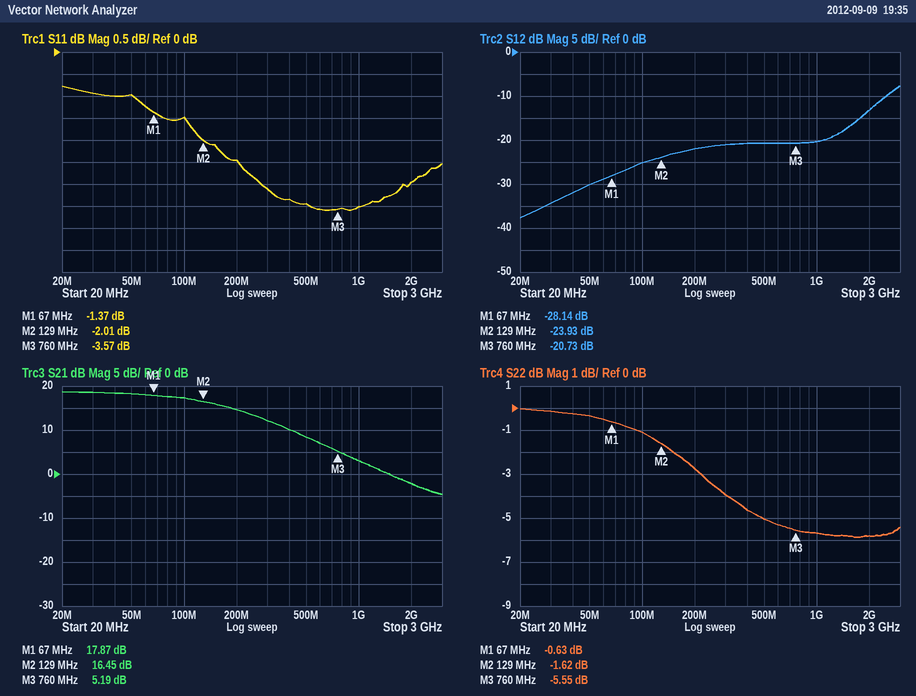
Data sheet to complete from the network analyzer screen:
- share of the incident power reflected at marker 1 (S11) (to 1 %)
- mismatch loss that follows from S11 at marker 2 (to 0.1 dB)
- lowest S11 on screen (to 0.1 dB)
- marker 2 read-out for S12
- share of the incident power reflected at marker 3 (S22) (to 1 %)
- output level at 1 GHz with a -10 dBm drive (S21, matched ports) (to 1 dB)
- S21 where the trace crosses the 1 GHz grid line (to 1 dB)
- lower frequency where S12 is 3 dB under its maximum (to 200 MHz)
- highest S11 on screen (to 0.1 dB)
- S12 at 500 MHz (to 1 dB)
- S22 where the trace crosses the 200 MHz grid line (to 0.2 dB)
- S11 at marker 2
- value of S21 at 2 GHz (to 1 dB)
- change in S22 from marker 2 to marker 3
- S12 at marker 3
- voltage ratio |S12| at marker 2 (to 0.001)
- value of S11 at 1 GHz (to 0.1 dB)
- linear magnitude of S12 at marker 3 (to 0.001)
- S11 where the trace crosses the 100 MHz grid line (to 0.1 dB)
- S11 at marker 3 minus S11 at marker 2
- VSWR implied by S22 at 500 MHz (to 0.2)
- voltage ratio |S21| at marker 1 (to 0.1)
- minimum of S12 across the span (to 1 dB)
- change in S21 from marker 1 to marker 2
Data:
73 %
4.3 dB
-3.6 dB
-23.93 dB
28 %
-7 dBm
3 dB
2.4 GHz
-0.8 dB
-21 dB
-2.8 dB
-2.01 dB
-2 dB
-3.93 dB
-20.73 dB
0.064
-3.5 dB
0.092
-1.5 dB
-1.56 dB
3.6
7.8
-38 dB
-1.42 dB
